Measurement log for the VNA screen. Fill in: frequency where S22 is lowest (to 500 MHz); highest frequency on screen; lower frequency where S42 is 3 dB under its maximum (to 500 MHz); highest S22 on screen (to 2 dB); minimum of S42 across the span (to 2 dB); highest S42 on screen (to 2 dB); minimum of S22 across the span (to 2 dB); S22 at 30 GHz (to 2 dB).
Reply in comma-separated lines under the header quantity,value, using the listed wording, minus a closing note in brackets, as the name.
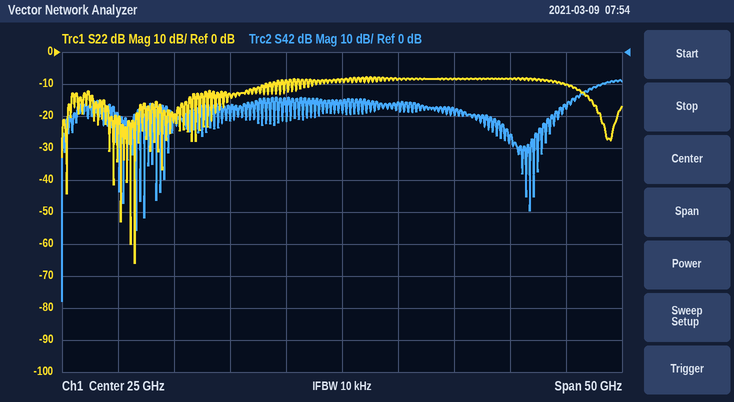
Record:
quantity,value
frequency where S22 is lowest,6.5 GHz
highest frequency on screen,50 GHz
lower frequency where S42 is 3 dB under its maximum,47.0 GHz
highest S22 on screen,-8 dB
minimum of S42 across the span,-78 dB
highest S42 on screen,-8 dB
minimum of S22 across the span,-66 dB
S22 at 30 GHz,-8 dB
